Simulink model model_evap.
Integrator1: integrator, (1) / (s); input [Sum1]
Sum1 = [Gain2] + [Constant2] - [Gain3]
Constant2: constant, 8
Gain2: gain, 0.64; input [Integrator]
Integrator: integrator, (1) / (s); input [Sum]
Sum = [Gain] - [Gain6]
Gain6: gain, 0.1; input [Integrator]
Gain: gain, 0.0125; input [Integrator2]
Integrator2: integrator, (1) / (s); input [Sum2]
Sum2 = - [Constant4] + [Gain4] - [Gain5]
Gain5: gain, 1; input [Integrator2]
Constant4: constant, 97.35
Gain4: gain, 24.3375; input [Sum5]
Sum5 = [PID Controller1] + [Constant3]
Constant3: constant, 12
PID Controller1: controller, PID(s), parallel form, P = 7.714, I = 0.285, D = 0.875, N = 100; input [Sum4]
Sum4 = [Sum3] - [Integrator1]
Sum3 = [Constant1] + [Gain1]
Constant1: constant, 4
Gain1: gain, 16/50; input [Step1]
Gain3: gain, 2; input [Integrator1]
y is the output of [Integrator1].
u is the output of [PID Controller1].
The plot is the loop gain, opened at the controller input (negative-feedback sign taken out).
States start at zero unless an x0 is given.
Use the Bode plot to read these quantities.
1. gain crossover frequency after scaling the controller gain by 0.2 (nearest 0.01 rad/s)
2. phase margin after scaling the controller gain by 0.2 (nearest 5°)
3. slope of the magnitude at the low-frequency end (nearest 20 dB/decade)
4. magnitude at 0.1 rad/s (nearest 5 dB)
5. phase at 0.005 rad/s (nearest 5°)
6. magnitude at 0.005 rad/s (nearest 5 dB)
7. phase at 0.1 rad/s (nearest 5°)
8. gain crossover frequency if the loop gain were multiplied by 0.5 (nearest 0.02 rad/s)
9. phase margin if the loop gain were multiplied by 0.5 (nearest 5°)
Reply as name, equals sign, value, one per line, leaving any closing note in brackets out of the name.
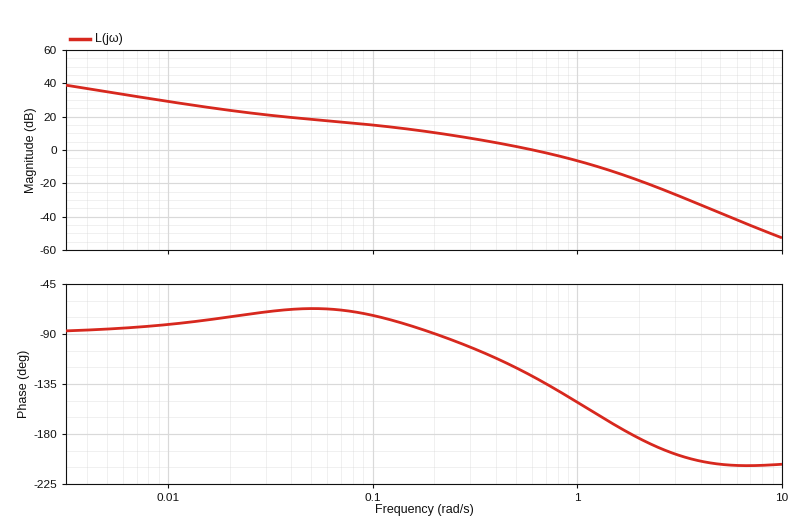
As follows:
gain crossover frequency after scaling the controller gain by 0.2 = 0.12 rad/s
phase margin after scaling the controller gain by 0.2 = 105°
slope of the magnitude at the low-frequency end = -20 dB/decade
magnitude at 0.1 rad/s = 15 dB
phase at 0.005 rad/s = -85°
magnitude at 0.005 rad/s = 35 dB
phase at 0.1 rad/s = -75°
gain crossover frequency if the loop gain were multiplied by 0.5 = 0.34 rad/s
phase margin if the loop gain were multiplied by 0.5 = 75°
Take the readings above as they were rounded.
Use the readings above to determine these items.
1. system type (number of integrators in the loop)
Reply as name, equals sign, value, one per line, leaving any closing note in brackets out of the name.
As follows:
system type = 1
